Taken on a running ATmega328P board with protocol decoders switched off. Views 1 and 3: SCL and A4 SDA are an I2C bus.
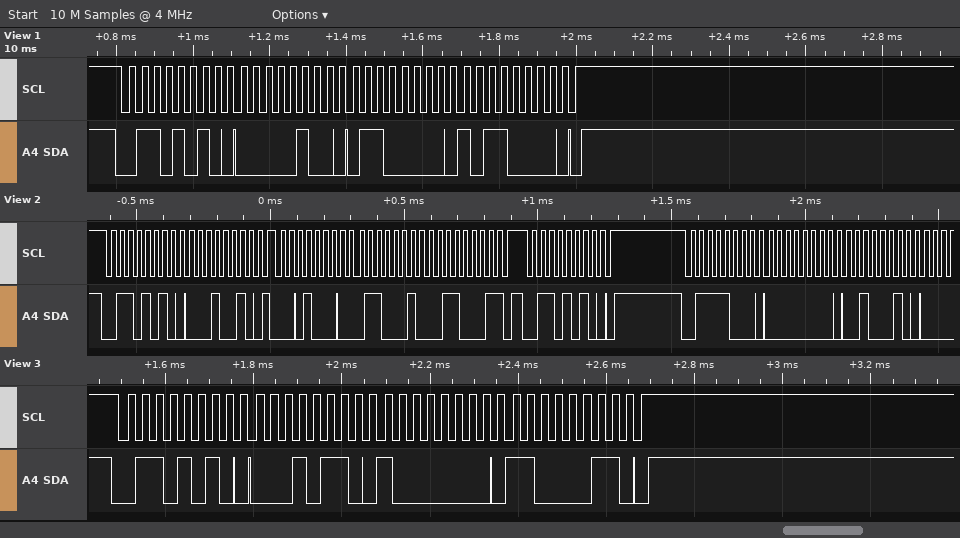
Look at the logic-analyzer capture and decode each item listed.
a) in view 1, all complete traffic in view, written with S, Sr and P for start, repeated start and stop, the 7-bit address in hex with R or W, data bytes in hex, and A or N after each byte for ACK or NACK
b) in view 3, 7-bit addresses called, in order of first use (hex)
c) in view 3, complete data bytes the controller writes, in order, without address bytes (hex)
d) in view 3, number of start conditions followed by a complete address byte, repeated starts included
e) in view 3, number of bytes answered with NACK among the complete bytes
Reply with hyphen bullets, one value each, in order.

- S 35W A 04 A 60 A B0 A P
- 0x35
- 16 80 C3
- 1
- 0
